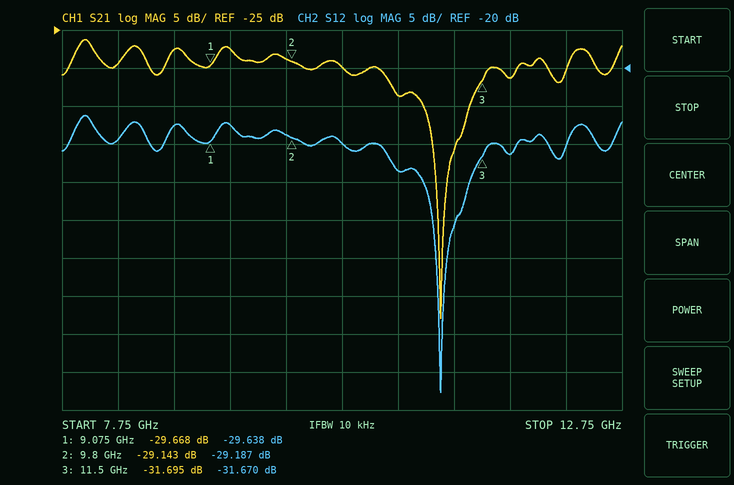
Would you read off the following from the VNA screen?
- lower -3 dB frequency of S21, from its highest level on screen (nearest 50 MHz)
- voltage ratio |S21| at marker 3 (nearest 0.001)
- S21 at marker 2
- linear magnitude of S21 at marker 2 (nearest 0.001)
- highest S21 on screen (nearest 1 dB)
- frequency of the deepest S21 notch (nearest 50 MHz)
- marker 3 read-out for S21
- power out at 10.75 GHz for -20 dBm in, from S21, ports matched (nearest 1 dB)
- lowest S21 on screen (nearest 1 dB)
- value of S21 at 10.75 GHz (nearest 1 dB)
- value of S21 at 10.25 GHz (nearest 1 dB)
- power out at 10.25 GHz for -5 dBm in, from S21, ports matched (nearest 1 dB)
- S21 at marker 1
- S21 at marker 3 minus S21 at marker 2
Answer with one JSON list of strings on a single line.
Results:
["7.85 GHz", "0.026", "-29.143 dB", "0.035", "-26 dB", "11.15 GHz", "-31.695 dB", "-54 dBm", "-63 dB", "-34 dB", "-30 dB", "-35 dBm", "-29.668 dB", "-2.552 dB"]
